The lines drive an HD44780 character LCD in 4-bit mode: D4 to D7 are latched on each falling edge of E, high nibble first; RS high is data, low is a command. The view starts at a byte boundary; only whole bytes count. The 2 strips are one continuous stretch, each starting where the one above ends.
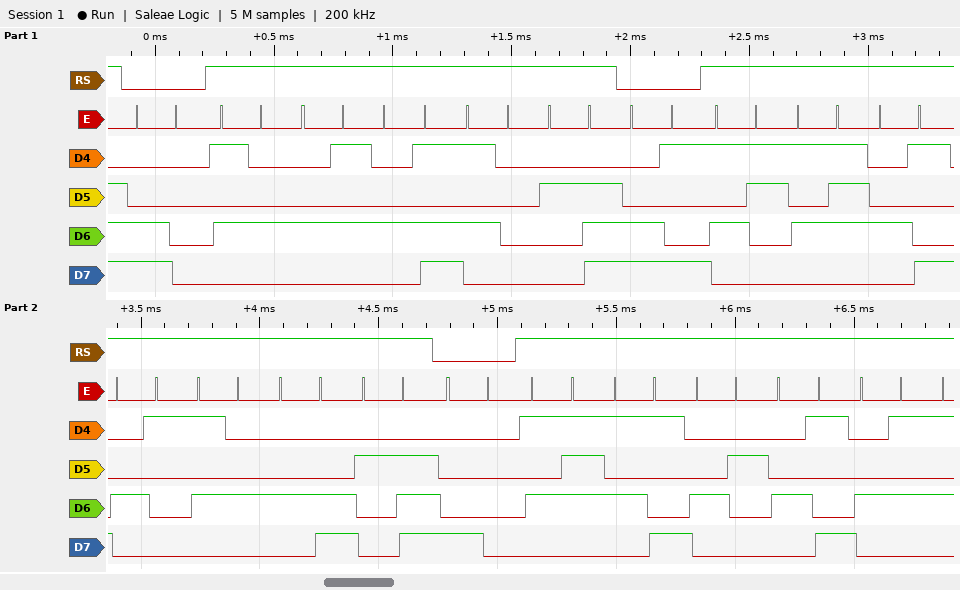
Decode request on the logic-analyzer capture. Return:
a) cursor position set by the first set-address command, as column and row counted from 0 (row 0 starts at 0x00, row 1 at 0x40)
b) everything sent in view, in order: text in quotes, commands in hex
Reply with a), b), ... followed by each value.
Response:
a) column 0, row 1
b) 0xC0 "TEMP." 0xC9 "SWIATL." 0x80 "WYBIE"
